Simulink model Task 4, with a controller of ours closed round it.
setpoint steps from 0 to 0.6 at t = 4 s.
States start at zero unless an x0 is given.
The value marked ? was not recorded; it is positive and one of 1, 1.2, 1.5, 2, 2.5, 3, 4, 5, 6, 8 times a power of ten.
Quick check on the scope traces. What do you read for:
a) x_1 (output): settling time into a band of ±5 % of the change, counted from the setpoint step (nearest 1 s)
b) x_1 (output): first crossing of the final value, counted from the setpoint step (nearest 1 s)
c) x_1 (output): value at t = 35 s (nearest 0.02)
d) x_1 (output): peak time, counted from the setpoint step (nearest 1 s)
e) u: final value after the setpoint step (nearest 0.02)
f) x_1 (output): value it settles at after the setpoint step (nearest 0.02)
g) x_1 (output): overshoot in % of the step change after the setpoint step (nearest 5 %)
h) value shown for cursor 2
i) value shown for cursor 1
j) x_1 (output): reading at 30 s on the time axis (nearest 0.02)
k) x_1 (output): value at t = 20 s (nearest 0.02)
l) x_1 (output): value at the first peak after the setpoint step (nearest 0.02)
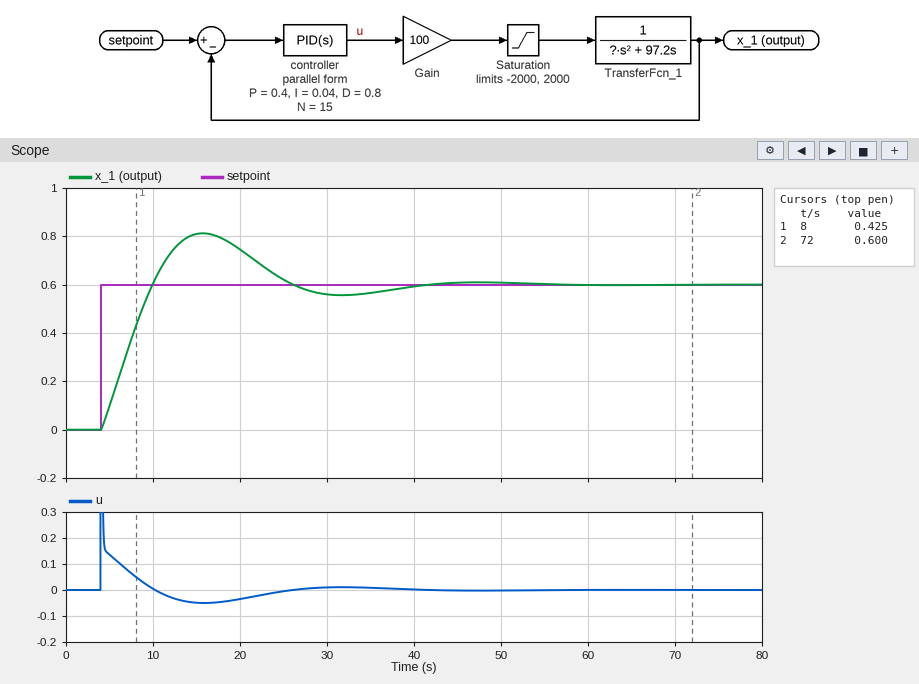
32 s
6 s
0.56
12 s
0.00
0.60
35 %
0.600
0.425
0.56
0.74
0.82
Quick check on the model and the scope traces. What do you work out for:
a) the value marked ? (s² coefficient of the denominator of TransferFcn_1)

500
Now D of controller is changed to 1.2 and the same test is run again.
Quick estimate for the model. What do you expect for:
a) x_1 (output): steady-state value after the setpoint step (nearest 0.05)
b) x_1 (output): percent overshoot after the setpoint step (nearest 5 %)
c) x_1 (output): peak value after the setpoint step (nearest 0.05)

0.60
25 %
0.75
